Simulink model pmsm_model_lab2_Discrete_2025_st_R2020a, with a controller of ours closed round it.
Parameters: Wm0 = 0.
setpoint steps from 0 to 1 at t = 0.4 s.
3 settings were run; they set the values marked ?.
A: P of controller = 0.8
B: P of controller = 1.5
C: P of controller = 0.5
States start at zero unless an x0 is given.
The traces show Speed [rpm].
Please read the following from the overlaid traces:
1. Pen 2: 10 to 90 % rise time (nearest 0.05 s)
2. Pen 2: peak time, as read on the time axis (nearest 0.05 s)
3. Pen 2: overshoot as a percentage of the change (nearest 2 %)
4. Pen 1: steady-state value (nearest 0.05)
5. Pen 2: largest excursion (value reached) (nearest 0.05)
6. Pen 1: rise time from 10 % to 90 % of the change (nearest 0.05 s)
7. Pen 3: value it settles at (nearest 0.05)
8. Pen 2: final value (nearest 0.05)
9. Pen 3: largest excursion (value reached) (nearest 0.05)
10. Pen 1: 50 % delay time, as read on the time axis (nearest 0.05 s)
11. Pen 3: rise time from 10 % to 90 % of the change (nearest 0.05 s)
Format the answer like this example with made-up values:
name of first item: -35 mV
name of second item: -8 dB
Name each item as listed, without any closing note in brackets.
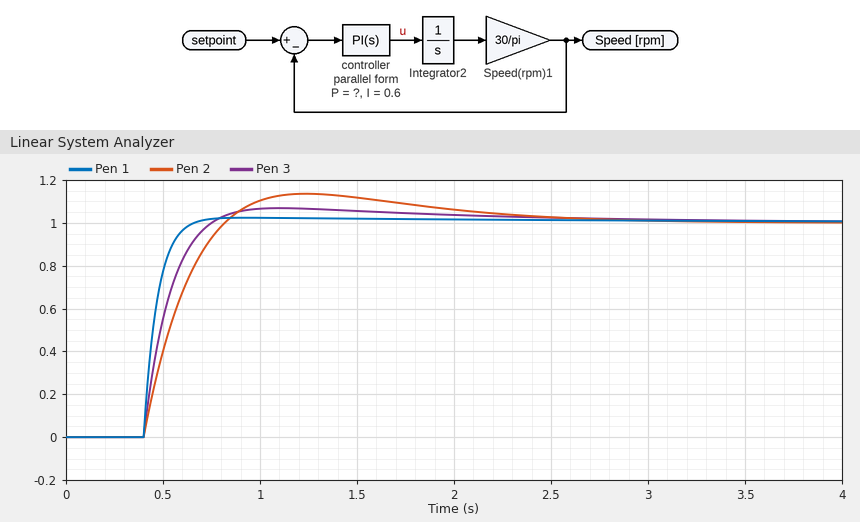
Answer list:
Pen 2: 10 to 90 % rise time: 0.30 s
Pen 2: peak time, as read on the time axis: 1.25 s
Pen 2: overshoot as a percentage of the change: 14 %
Pen 1: steady-state value: 1.00
Pen 2: largest excursion (value reached): 1.15
Pen 1: rise time from 10 % to 90 % of the change: 0.15 s
Pen 3: value it settles at: 1.00
Pen 2: final value: 1.00
Pen 3: largest excursion (value reached): 1.05
Pen 1: 50 % delay time, as read on the time axis: 0.45 s
Pen 3: rise time from 10 % to 90 % of the change: 0.25 s
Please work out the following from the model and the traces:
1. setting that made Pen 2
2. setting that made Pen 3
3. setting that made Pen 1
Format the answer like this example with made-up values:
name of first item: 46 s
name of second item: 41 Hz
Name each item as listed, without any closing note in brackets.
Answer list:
setting that made Pen 2: C
setting that made Pen 3: A
setting that made Pen 1: B
